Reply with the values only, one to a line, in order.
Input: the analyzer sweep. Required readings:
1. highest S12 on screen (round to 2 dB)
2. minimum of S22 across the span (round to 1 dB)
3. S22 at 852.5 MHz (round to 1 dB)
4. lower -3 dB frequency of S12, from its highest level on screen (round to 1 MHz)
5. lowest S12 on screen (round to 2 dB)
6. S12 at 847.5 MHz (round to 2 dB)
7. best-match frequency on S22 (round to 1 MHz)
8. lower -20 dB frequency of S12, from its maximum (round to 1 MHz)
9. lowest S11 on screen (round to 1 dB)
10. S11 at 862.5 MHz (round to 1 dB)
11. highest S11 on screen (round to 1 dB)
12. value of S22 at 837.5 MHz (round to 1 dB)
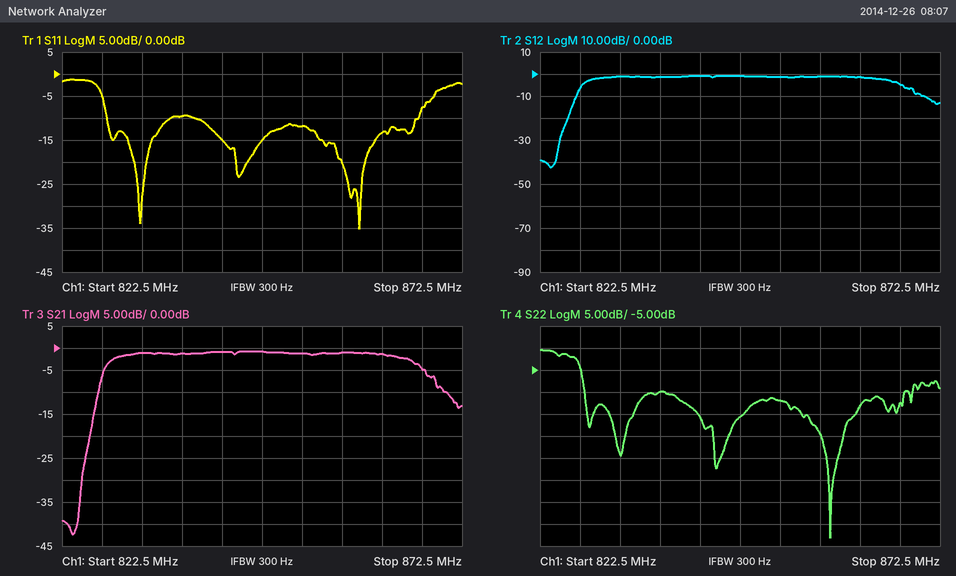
0 dB
-43 dB
-12 dB
828 MHz
-42 dB
0 dB
859 MHz
826 MHz
-35 dB
-13 dB
-1 dB
-10 dB
